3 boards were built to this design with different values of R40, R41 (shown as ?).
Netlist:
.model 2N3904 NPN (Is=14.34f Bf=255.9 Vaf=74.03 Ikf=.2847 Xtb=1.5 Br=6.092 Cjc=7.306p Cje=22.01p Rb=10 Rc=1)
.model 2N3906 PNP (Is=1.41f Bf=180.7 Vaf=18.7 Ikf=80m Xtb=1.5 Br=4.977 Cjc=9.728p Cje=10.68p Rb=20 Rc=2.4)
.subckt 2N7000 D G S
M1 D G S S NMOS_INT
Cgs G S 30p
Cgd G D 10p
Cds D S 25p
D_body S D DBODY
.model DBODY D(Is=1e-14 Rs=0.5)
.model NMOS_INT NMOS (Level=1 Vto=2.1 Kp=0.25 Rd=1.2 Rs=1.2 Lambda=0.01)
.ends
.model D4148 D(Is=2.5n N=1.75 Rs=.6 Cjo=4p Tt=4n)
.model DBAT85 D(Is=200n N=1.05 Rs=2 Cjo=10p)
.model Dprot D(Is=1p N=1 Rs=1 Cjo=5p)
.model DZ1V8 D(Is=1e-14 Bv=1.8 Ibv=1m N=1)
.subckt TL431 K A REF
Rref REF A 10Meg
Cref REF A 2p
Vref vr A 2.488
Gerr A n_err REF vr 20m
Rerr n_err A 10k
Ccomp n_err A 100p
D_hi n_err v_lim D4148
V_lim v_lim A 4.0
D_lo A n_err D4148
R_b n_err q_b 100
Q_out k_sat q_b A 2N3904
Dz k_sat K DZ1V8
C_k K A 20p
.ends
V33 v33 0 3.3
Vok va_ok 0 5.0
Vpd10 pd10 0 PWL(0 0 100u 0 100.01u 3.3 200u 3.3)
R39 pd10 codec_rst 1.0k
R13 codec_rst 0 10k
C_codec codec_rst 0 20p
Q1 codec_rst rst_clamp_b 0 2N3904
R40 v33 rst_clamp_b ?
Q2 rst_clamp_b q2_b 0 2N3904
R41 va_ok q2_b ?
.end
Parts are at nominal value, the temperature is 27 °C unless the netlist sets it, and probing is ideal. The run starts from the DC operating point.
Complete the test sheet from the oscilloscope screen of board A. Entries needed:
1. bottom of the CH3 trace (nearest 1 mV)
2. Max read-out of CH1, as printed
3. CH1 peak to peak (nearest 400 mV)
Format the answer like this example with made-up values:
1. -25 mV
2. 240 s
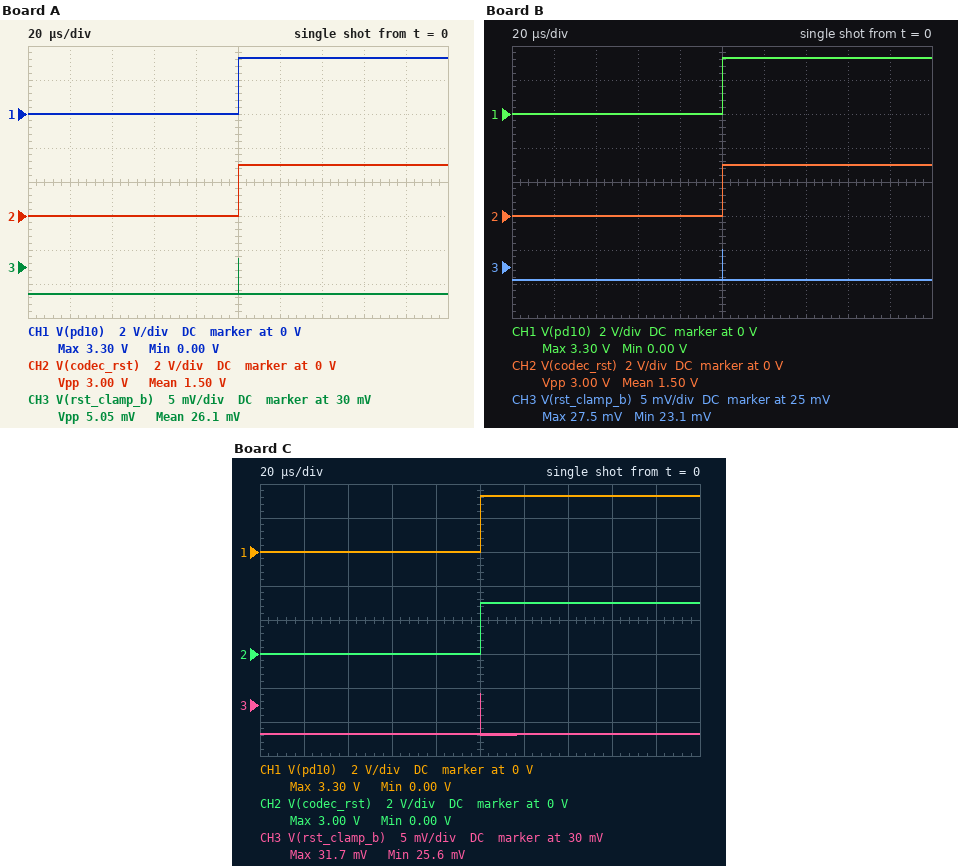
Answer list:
1. 26 mV
2. 3.30 V
3. 3.2 V
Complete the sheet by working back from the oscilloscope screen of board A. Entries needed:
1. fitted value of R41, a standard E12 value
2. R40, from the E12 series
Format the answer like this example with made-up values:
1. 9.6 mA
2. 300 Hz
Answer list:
1. 15 kΩ
2. 1.5 kΩ
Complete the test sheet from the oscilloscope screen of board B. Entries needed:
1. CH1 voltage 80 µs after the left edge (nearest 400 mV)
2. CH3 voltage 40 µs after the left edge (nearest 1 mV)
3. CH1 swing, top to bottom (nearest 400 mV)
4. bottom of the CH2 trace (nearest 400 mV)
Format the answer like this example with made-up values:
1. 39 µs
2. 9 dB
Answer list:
1. 0 V
2. 23 mV
3. 3.2 V
4. 0 V
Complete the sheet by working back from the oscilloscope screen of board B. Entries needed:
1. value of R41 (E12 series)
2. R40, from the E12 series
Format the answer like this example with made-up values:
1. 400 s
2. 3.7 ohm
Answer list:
1. 12 kΩ
2. 1.5 kΩ
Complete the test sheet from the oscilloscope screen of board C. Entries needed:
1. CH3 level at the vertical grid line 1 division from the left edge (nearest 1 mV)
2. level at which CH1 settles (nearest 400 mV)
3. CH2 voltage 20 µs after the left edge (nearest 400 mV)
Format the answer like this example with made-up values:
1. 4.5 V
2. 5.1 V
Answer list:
1. 26 mV
2. 3.2 V
3. 0 V
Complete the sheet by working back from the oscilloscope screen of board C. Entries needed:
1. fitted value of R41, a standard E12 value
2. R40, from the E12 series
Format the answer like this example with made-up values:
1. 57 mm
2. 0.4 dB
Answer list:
1. 18 kΩ
2. 1.8 kΩ
